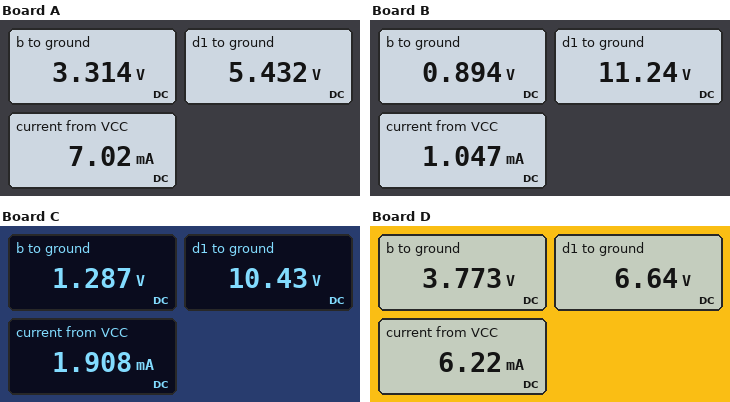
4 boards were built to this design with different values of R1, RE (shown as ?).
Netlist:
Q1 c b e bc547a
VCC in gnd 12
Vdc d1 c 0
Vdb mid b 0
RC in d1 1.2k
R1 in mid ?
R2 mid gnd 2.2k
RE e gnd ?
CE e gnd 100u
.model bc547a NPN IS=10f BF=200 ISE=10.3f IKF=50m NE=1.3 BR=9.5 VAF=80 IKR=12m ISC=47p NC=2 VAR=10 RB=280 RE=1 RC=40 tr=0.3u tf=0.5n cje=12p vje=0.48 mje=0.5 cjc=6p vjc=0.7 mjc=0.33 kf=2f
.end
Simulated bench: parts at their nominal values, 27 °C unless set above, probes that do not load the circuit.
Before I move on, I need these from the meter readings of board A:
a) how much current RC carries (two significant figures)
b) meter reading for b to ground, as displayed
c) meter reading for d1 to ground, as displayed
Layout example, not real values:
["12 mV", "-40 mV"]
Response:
["5.5 mA", "3.314 V", "5.432 V"]
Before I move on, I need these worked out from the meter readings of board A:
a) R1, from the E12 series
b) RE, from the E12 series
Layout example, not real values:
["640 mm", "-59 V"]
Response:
["5.6 kΩ", "470 Ω"]
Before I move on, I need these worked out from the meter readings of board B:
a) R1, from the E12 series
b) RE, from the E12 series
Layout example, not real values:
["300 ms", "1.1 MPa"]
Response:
["27 kΩ", "390 Ω"]
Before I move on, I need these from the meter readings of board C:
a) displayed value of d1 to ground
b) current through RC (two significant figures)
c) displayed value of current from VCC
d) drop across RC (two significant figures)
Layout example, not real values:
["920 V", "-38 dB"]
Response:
["10.43 V", "1.3 mA", "1.908 mA", "1.6 V"]
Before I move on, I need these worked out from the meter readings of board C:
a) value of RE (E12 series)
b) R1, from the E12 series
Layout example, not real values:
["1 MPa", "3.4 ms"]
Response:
["470 Ω", "18 kΩ"]
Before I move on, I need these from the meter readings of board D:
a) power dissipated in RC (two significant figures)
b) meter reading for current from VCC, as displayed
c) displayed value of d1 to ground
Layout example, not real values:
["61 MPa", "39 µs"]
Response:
["24 mW", "6.22 mA", "6.64 V"]
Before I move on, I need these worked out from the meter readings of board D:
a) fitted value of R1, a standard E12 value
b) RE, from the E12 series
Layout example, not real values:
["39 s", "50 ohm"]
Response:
["4.7 kΩ", "680 Ω"]
